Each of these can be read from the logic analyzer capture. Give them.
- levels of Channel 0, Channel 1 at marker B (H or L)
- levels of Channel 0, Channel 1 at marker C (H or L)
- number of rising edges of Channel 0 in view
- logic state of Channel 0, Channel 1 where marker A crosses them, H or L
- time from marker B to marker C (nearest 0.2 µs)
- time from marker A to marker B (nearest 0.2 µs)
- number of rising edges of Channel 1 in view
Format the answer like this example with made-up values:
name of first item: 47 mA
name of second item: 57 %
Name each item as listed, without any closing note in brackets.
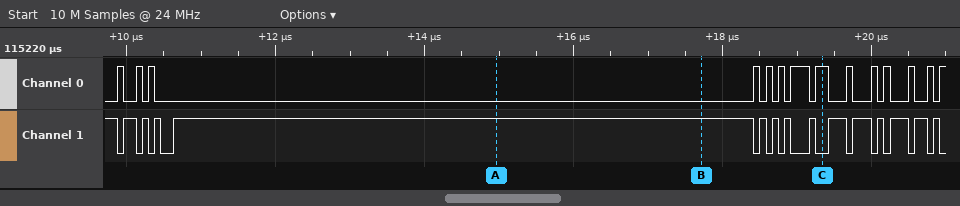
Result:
levels of Channel 0, Channel 1 at marker B: Channel 0=L, Channel 1=H
levels of Channel 0, Channel 1 at marker C: Channel 0=H, Channel 1=L
number of rising edges of Channel 0 in view: 14
logic state of Channel 0, Channel 1 where marker A crosses them, H or L: Channel 0=L, Channel 1=H
time from marker B to marker C: 1.6 µs
time from marker A to marker B: 2.8 µs
number of rising edges of Channel 1 in view: 14
